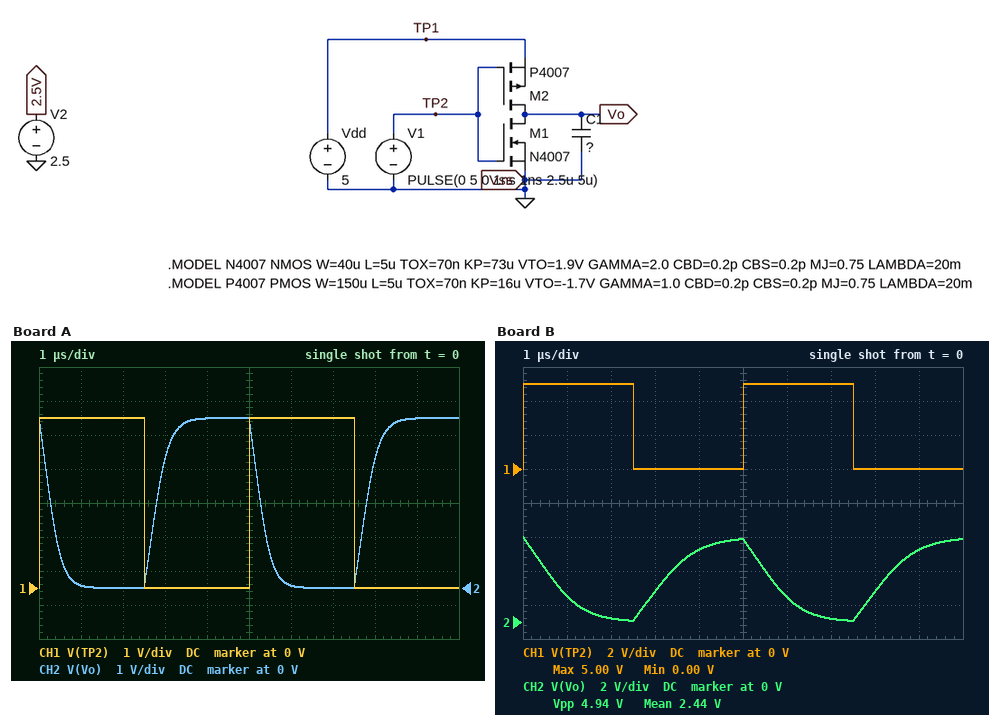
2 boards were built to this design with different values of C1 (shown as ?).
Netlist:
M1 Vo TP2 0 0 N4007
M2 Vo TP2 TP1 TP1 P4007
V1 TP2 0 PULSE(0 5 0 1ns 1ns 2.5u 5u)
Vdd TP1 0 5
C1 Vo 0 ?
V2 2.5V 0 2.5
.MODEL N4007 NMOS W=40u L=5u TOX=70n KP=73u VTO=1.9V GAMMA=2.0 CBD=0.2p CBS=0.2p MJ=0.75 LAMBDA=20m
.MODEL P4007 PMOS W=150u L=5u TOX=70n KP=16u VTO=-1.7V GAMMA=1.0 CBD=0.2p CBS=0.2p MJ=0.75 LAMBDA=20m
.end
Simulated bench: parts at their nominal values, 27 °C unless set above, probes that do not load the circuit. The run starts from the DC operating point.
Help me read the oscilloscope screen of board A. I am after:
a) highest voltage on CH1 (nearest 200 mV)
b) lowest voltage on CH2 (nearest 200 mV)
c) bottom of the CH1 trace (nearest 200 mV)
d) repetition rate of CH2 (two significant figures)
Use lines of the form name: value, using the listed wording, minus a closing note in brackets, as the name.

highest voltage on CH1: 5.0 V
lowest voltage on CH2: 0 V
bottom of the CH1 trace: 0 V
repetition rate of CH2: 200 kHz
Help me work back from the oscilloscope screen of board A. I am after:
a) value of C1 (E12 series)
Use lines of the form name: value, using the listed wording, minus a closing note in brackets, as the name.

value of C1: 330 pF
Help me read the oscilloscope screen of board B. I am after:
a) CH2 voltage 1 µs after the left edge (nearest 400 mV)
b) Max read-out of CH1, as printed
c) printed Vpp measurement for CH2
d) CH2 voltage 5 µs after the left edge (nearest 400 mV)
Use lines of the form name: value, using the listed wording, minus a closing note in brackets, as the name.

CH2 voltage 1 µs after the left edge: 1.6 V
Max read-out of CH1, as printed: 5.00 V
printed Vpp measurement for CH2: 4.94 V
CH2 voltage 5 µs after the left edge: 4.8 V
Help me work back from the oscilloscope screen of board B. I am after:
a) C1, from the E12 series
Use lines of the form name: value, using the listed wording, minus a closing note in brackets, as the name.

C1, from the E12 series: 820 pF
